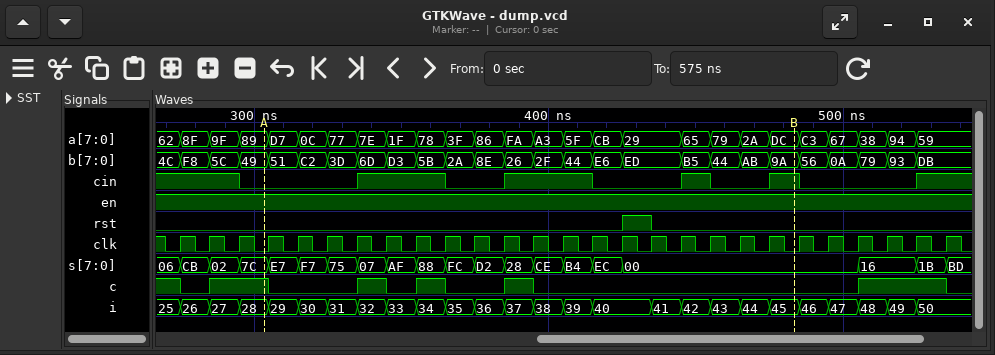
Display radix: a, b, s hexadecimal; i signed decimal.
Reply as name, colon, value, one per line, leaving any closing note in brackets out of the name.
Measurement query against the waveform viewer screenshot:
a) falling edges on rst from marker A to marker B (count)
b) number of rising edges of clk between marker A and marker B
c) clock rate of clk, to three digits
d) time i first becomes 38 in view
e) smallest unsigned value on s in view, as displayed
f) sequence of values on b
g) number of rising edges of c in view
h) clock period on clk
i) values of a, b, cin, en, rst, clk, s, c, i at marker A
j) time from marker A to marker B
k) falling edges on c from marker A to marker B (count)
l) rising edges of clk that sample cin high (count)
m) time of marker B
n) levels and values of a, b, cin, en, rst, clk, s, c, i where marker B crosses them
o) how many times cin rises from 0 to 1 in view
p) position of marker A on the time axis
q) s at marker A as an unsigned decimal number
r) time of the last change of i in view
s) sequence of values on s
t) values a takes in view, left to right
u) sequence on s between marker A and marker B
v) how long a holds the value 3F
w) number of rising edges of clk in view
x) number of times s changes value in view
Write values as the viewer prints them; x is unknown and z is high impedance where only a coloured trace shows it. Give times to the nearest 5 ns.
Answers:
falling edges on rst from marker A to marker B: 1
number of rising edges of clk between marker A and marker B: 18
clock rate of clk, to three digits: 100 MHz
time i first becomes 38 in view: 395 ns
smallest unsigned value on s in view, as displayed: 00
sequence of values on b: 4C, F8, 5C, 49, 51, C2, 3D, 6D, D3, 5B, 2A, 8E, 26, 2F, 44, E6, ED, B5, 44, AB, 9A, 56, 0A, 79, 93, DB
number of rising edges of c in view: 5
clock period on clk: 10 ns
values of a, b, cin, en, rst, clk, s, c, i at marker A: a=89, b=49, cin=0, en=1, rst=0, clk=0, s=7C, c=1, i=28
time from marker A to marker B: 180 ns
falling edges on c from marker A to marker B: 4
rising edges of clk that sample cin high: 12
time of marker B: 485 ns
levels and values of a, b, cin, en, rst, clk, s, c, i where marker B crosses them: a=DC, b=9A, cin=1, en=1, rst=0, clk=0, s=00, c=0, i=45
how many times cin rises from 0 to 1 in view: 5
position of marker A on the time axis: 305 ns
s at marker A as an unsigned decimal number: 124
time of the last change of i in view: 525 ns
sequence of values on s: 06, CB, 02, 7C, E7, F7, 75, 07, AF, 88, FC, D2, 28, CE, B4, EC, 00, 16, 1B, BD
values a takes in view, left to right: 62, 8F, 9F, 89, D7, 0C, 77, 7E, 1F, 78, 3F, 86, FA, A3, 5F, CB, 29, 65, 79, 2A, DC, C3, 67, 38, 94, 59
sequence on s between marker A and marker B: 7C, E7, F7, 75, 07, AF, 88, FC, D2, 28, CE, B4, EC, 00
how long a holds the value 3F: 10 ns
number of rising edges of clk in view: 27
number of times s changes value in view: 19
